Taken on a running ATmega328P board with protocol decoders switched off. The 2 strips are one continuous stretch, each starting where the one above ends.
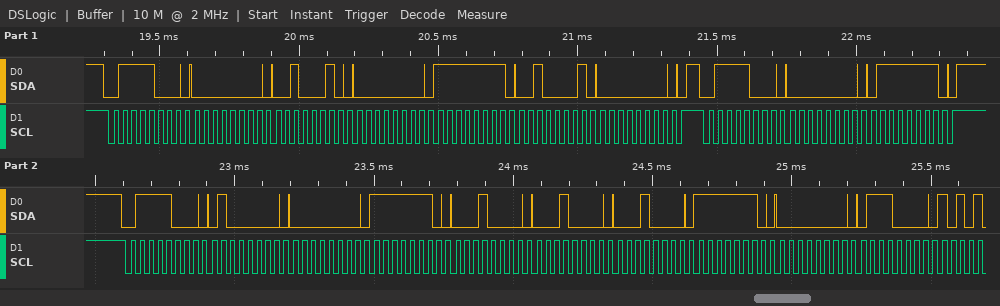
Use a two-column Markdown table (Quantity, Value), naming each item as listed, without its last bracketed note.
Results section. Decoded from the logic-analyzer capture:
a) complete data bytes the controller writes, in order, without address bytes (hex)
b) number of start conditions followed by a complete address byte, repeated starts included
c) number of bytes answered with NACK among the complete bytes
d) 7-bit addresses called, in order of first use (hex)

| Quantity | Value |
|---|---|
| complete data bytes the controller writes, in order, without address bytes | 00 22 00 FF 21 00 00 7F 40 00 FE 10 10 10 FE 00 70 |
| number of start conditions followed by a complete address byte, repeated starts included | 3 |
| number of bytes answered with NACK among the complete bytes | 0 |
| 7-bit addresses called, in order of first use | 0x3C |
